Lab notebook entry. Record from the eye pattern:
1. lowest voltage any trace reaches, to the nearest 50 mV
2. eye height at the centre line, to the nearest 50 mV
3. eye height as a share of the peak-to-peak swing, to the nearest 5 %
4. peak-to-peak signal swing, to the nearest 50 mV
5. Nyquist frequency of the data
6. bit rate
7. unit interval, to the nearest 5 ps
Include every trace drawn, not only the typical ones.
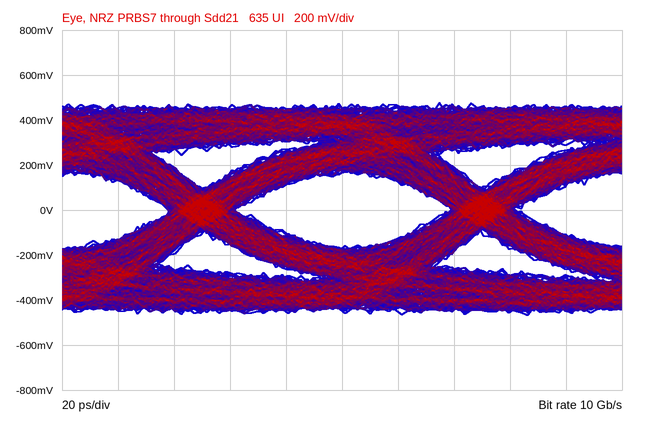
-450 mV
350 mV
35 %
950 mV
5 GHz
10 Gb/s
100 ps
